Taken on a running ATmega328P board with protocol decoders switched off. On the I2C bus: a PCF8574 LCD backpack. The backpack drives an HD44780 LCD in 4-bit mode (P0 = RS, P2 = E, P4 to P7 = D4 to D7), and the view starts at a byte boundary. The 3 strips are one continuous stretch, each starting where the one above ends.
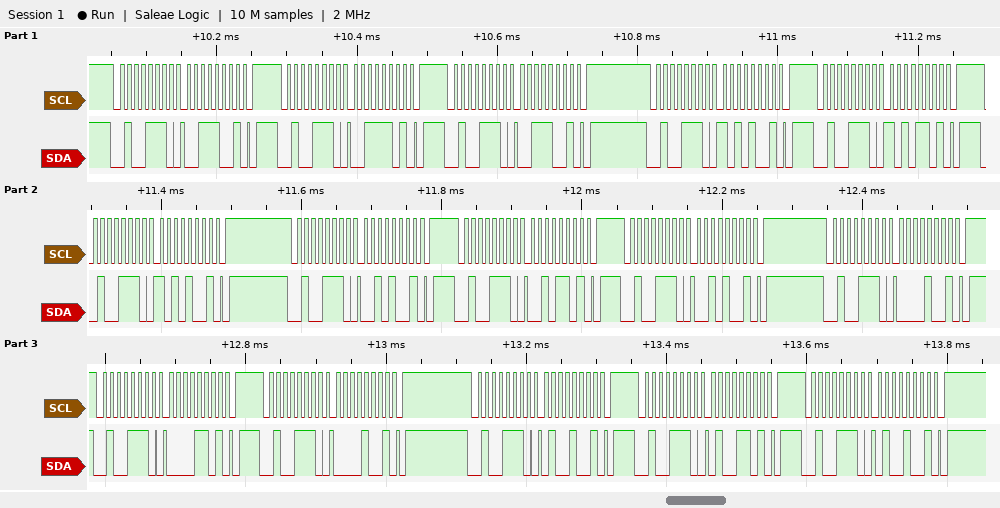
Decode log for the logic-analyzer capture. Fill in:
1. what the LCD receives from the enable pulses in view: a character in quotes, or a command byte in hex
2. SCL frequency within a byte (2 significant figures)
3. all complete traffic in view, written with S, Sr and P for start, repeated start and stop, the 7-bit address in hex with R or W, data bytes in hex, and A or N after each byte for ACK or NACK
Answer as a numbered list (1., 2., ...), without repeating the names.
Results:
1. ':' ' '
2. 100 kHz
3. S 27W A 39 A P S 27W A 3D A P S 27W A 39 A P S 27W A A9 A P S 27W A AD A P S 27W A A9 A P S 27W A 29 A P S 27W A 2D A P S 27W A 29 A P S 27W A 09 A P S 27W A 0D A P S 27W A 09 A P S 27W A 49 A P S 27W A 4D A P S 27W A 49 A P
